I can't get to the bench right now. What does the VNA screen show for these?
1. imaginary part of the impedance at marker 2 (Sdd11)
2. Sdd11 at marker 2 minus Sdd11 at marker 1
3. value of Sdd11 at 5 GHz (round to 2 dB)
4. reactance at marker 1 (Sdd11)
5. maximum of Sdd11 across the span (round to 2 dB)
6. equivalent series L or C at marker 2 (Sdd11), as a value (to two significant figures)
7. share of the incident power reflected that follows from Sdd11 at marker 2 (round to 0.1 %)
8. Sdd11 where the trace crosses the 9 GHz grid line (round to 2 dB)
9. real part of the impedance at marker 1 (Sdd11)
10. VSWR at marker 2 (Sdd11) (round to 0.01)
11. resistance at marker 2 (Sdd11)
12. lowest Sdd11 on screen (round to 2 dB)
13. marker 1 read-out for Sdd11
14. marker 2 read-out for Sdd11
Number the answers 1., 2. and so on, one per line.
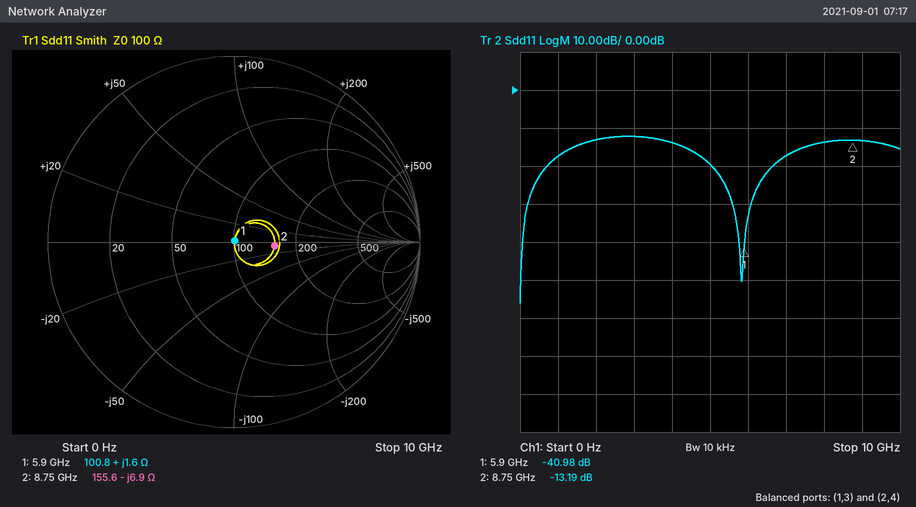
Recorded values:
1. -6.9 Ω
2. 27.79 dB
3. -20 dB
4. +1.6 Ω
5. -12 dB
6. 2.6 pF
7. 4.8 %
8. -14 dB
9. 100.8 Ω
10. 1.56
11. 155.6 Ω
12. -56 dB
13. -40.98 dB
14. -13.19 dB
